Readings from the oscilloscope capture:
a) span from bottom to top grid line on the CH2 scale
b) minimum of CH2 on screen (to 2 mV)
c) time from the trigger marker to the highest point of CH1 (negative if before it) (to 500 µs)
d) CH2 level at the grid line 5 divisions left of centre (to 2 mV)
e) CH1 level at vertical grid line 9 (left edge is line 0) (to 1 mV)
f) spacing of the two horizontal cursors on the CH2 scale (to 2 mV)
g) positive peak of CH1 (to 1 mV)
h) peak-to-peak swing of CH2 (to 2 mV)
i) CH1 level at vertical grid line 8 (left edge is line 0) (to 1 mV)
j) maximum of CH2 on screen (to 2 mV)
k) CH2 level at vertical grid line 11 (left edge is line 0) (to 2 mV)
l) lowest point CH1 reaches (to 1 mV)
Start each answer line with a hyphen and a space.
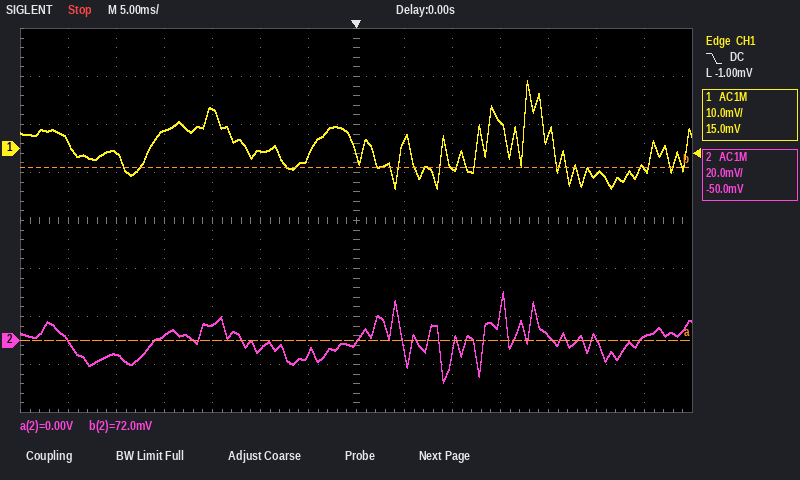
- 160 mV
- -18 mV
- +18.0 ms
- -6 mV
- -4 mV
- 72 mV
- 14 mV
- 38 mV
- 2 mV
- 20 mV
- 2 mV
- -8 mV
